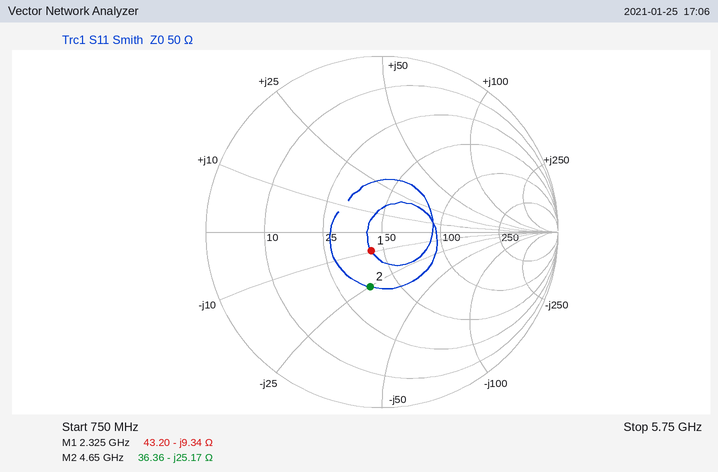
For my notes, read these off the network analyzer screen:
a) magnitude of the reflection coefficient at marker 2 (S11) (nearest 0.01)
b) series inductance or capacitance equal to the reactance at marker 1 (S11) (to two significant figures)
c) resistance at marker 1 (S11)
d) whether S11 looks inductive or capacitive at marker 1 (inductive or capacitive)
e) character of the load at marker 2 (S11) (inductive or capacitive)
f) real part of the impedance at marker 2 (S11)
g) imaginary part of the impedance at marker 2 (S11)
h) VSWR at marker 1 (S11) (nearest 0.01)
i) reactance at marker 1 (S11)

0.32
7.3 pF
43.20 Ω
capacitive
capacitive
36.36 Ω
-25.17 Ω
1.28
-9.34 Ω
